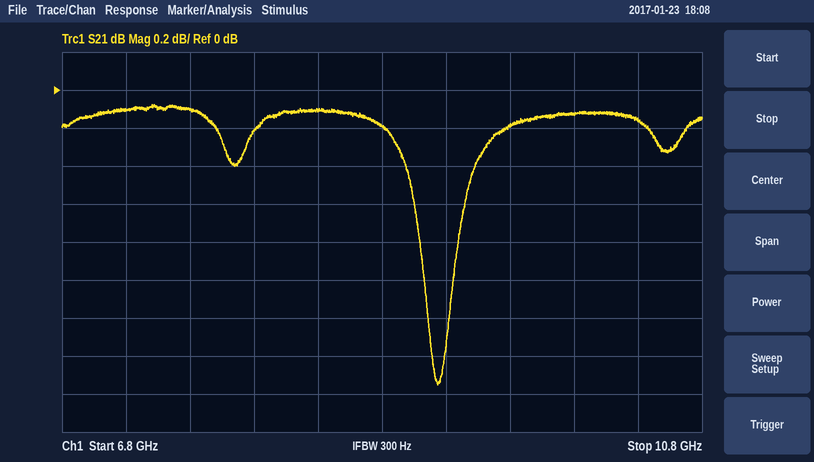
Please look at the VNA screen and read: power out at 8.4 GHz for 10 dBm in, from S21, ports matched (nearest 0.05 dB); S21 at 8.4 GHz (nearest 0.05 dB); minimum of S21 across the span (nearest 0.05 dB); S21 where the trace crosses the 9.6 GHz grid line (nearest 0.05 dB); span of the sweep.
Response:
9.90 dBm
-0.10 dB
-1.55 dB
-0.20 dB
4 GHz
